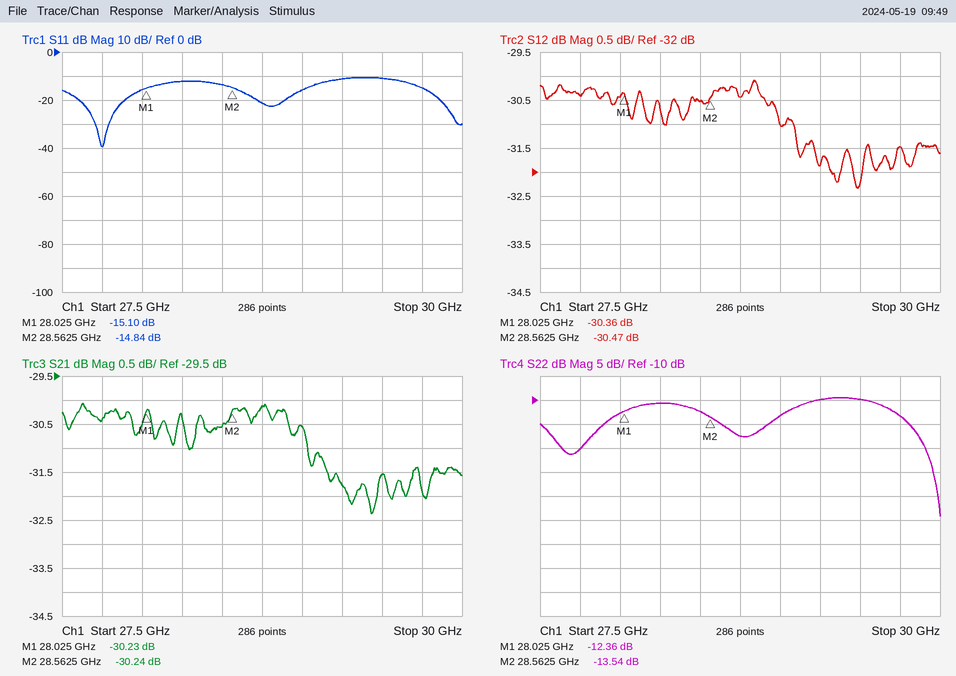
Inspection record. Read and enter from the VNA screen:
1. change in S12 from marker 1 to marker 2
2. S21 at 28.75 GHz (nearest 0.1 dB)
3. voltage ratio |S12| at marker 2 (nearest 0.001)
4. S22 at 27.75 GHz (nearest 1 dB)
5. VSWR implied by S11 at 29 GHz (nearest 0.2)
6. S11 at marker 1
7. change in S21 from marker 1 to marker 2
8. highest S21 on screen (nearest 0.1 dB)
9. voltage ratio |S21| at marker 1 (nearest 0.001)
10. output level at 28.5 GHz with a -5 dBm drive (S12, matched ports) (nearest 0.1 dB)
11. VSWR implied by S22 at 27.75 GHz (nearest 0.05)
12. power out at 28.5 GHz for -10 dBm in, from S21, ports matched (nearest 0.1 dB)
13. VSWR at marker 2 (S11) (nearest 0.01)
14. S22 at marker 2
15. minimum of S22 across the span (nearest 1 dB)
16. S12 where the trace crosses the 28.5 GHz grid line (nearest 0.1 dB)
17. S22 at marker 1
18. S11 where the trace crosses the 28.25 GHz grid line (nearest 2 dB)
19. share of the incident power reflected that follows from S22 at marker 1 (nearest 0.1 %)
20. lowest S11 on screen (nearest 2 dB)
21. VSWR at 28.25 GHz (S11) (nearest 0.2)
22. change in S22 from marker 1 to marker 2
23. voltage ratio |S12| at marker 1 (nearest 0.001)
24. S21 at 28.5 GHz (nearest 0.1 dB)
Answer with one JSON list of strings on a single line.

["-0.11 dB", "-30.1 dB", "0.030", "-20 dB", "1.4", "-15.10 dB", "-0.01 dB", "-30.1 dB", "0.031", "-35.5 dBm", "1.20", "-40.5 dBm", "1.44", "-13.54 dB", "-34 dB", "-30.5 dB", "-12.36 dB", "-12 dB", "5.8 %", "-40 dB", "1.6", "-1.18 dB", "0.030", "-30.5 dB"]
